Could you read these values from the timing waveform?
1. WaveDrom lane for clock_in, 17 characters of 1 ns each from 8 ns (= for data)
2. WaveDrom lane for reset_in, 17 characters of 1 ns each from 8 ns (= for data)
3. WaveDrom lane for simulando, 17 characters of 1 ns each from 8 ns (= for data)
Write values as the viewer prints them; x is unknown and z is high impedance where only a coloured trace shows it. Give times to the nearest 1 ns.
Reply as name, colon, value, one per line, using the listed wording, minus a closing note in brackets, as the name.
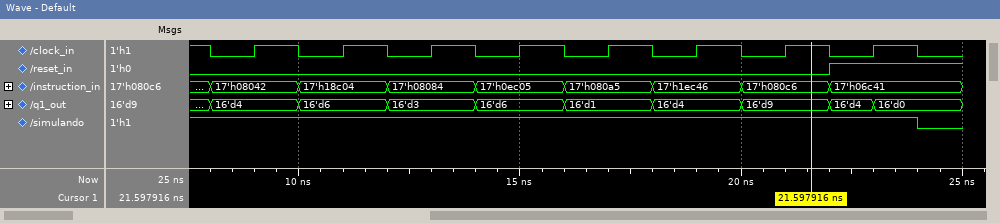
WaveDrom lane for clock_in, 17 characters of 1 ns each from 8 ns: {name: 'clock_in', wave: '01010101010101010'}
WaveDrom lane for reset_in, 17 characters of 1 ns each from 8 ns: {name: 'reset_in', wave: '0.............1..'}
WaveDrom lane for simulando, 17 characters of 1 ns each from 8 ns: {name: 'simulando', wave: '1...............0'}
